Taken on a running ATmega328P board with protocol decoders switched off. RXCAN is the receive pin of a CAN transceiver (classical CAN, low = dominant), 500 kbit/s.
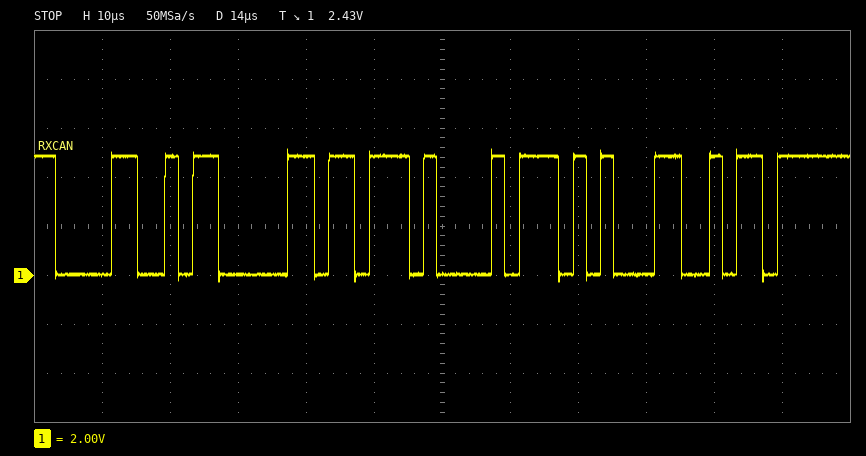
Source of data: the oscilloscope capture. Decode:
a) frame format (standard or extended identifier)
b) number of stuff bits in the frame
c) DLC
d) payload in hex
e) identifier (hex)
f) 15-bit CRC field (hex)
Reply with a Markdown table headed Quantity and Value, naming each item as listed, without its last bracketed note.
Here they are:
| Quantity | Value |
|---|---|
| frame format | standard |
| number of stuff bits in the frame | 1 |
| DLC | 2 |
| payload in hex | DD 0B |
| identifier | 0x0CB |
| 15-bit CRC field | 0x5465 |
